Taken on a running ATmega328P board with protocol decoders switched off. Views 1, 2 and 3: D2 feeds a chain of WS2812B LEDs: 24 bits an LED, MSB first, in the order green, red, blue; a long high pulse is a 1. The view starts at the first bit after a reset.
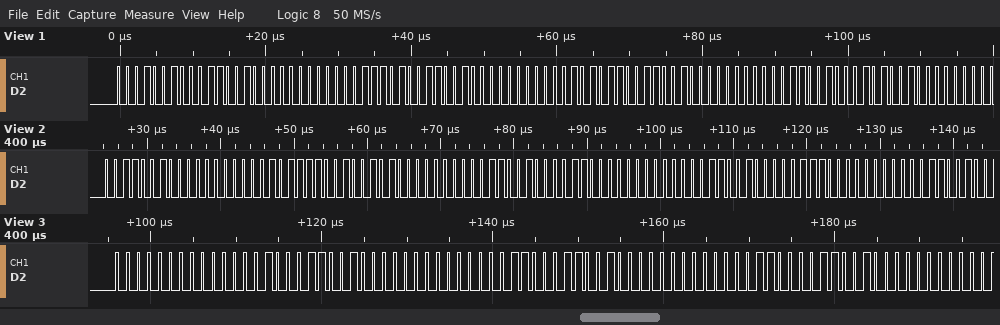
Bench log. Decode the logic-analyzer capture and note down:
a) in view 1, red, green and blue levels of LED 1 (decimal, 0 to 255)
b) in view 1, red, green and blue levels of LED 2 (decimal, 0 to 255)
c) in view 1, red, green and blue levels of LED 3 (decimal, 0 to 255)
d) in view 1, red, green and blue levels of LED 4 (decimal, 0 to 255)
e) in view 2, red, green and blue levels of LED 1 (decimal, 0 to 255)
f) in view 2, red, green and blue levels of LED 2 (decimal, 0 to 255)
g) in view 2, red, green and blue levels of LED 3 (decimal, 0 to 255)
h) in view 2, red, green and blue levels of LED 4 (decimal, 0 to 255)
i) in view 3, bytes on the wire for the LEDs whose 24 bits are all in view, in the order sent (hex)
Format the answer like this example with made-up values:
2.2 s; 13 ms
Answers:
50, 18, 0; 50, 29, 0; 50, 43, 0; 41, 50, 0; 0, 50, 47; 0, 37, 50; 0, 24, 50; 0, 14, 50; 00 02 32 00 06 32 00 0C 32
